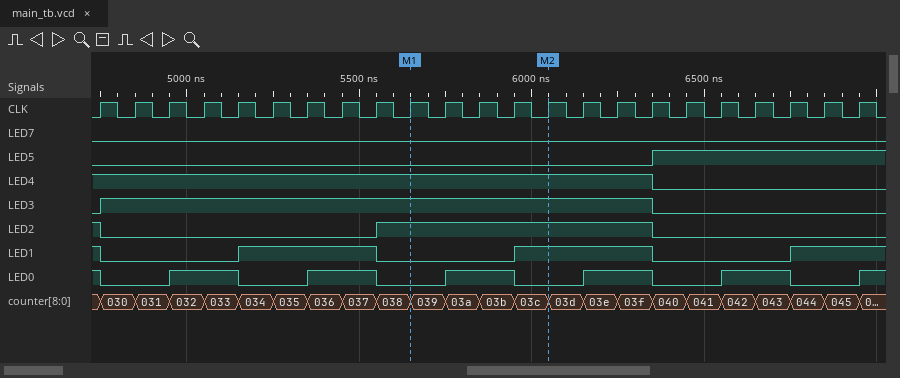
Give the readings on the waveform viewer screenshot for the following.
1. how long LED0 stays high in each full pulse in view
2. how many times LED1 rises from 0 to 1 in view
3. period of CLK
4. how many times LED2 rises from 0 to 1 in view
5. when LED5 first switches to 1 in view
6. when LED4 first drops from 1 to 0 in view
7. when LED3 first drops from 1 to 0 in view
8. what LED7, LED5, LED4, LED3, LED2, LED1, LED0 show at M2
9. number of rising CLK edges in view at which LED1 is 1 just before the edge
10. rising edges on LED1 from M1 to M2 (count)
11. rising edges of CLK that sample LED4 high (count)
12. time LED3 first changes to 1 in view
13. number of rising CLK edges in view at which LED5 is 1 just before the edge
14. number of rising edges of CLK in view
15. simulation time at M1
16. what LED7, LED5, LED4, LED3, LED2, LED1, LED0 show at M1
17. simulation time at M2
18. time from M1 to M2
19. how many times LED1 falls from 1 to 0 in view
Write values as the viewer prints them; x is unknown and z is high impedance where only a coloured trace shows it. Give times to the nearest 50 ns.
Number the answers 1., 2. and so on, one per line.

1. 200 ns, 200 ns, 200 ns, 200 ns, 200 ns
2. 3
3. 100 ns
4. 1
5. 6350 ns
6. 6350 ns
7. 6350 ns
8. LED7=0, LED5=0, LED4=1, LED3=1, LED2=1, LED1=1, LED0=0
9. 11
10. 1
11. 17
12. 4750 ns
13. 6
14. 23
15. 5650 ns
16. LED7=0, LED5=0, LED4=1, LED3=1, LED2=1, LED1=0, LED0=0
17. 6050 ns
18. 400 ns
19. 3
